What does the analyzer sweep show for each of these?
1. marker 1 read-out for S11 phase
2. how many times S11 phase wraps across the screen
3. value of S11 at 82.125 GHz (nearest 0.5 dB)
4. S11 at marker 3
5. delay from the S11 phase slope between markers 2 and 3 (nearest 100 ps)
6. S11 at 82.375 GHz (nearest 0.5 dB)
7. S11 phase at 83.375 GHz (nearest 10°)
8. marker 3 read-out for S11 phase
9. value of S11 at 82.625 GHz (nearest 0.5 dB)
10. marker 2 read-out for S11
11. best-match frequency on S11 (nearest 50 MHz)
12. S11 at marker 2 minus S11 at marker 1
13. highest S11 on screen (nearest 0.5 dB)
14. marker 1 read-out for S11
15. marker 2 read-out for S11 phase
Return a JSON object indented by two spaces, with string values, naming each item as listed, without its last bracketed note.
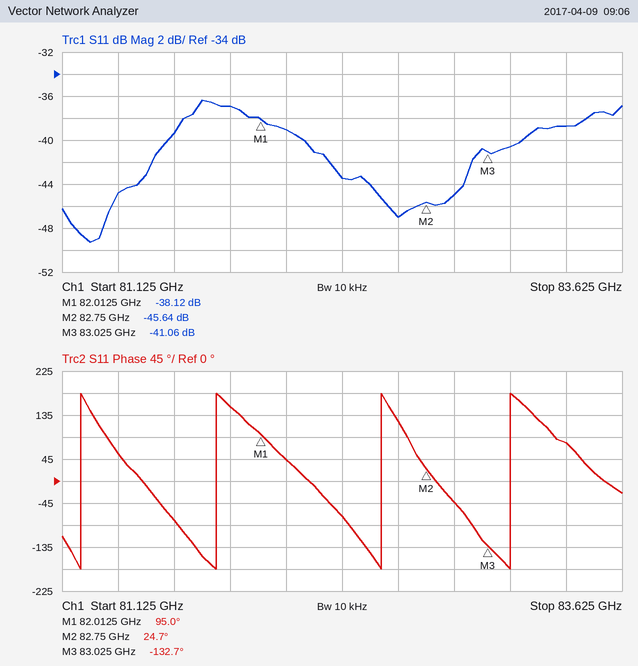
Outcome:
{
  "marker 1 read-out for S11 phase": "95.0°",
  "how many times S11 phase wraps across the screen": "4",
  "value of S11 at 82.125 GHz": "-39.0 dB",
  "S11 at marker 3": "-41.06 dB",
  "delay from the S11 phase slope between markers 2 and 3": "1.6 ns",
  "S11 at 82.375 GHz": "-43.5 dB",
  "S11 phase at 83.375 GHz": "80°",
  "marker 3 read-out for S11 phase": "-132.7°",
  "value of S11 at 82.625 GHz": "-47.0 dB",
  "marker 2 read-out for S11": "-45.64 dB",
  "best-match frequency on S11": "81.25 GHz",
  "S11 at marker 2 minus S11 at marker 1": "-7.52 dB",
  "highest S11 on screen": "-36.5 dB",
  "marker 1 read-out for S11": "-38.12 dB",
  "marker 2 read-out for S11 phase": "24.7°"
}
